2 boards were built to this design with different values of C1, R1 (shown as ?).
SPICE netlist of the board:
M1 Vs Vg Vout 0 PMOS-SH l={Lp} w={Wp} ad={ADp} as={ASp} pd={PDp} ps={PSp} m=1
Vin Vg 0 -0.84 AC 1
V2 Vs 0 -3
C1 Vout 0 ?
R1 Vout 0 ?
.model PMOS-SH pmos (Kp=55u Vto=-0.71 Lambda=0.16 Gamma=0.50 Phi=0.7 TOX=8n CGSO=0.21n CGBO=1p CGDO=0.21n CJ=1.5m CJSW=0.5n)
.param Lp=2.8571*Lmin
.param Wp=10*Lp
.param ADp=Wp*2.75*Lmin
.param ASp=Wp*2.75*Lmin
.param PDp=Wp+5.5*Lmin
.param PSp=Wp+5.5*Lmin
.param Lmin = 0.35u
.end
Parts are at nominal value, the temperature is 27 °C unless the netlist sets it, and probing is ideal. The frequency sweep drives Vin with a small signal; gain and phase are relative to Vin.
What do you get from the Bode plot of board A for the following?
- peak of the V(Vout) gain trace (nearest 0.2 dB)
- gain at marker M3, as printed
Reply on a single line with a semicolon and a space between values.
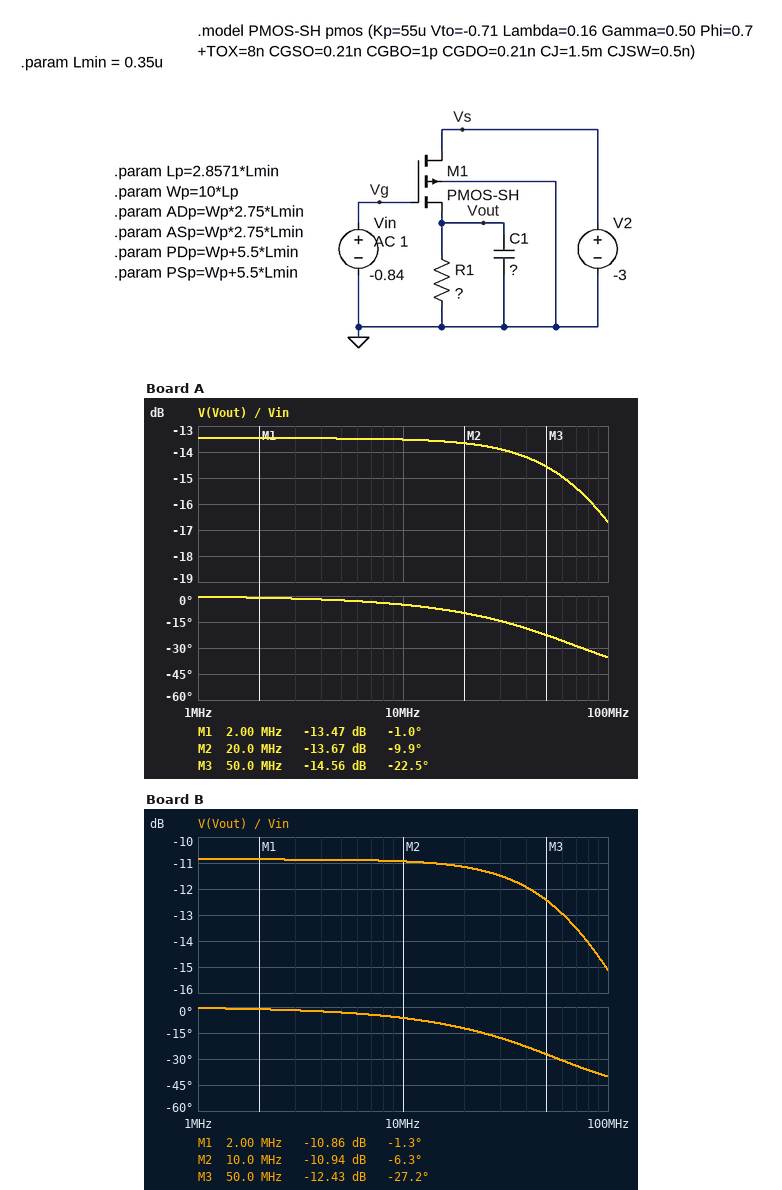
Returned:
-13.4 dB; -14.56 dB
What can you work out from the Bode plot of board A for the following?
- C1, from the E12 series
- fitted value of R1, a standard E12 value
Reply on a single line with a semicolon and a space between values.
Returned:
680 fF; 3.3 kΩ
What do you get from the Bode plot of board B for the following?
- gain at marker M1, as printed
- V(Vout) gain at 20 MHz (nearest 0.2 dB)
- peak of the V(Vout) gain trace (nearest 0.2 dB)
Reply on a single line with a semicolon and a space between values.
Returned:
-10.86 dB; -11.2 dB; -10.8 dB
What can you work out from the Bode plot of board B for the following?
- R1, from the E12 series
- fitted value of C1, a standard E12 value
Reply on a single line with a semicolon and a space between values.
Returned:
5.6 kΩ; 560 fF
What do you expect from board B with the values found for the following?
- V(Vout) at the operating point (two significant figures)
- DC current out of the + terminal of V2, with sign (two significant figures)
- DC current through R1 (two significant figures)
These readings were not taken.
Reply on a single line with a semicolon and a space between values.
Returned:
-23 mV; -4.1 µA; 4.1 µA
